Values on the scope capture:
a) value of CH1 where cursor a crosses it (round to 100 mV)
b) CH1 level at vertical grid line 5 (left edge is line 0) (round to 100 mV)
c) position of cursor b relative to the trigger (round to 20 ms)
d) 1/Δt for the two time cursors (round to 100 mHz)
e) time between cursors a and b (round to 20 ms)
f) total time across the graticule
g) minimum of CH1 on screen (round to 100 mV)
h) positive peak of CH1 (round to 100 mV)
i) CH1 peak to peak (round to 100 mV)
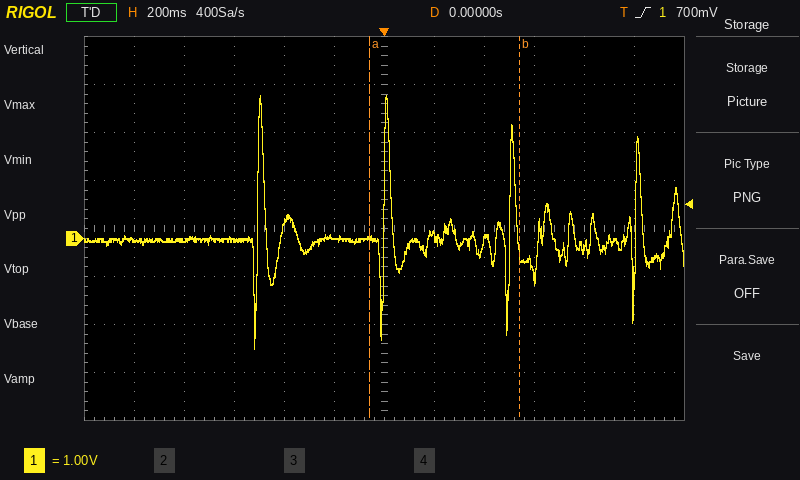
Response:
0.0 V
0.0 V
+540 ms
1.7 Hz
600 ms
2.4 s
-2.3 V
3.0 V
5.3 V
